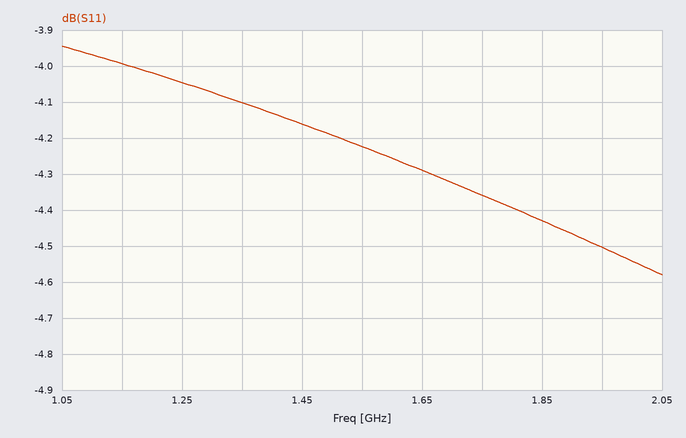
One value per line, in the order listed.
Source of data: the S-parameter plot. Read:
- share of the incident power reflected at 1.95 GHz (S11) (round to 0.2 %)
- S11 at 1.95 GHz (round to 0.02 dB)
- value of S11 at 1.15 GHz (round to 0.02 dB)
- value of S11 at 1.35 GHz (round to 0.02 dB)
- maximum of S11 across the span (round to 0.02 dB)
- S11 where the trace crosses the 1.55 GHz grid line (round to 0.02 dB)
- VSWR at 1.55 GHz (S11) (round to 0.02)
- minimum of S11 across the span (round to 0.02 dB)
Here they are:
35.4 %
-4.50 dB
-4.00 dB
-4.10 dB
-3.94 dB
-4.22 dB
4.20
-4.58 dB
